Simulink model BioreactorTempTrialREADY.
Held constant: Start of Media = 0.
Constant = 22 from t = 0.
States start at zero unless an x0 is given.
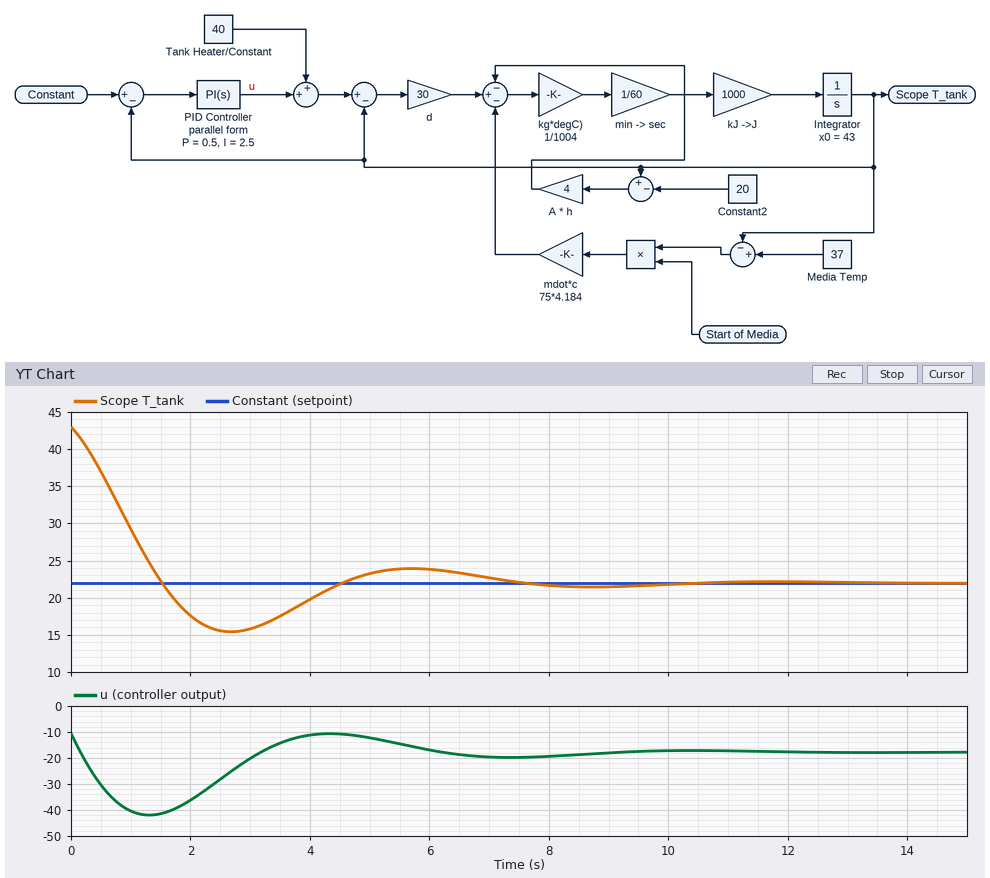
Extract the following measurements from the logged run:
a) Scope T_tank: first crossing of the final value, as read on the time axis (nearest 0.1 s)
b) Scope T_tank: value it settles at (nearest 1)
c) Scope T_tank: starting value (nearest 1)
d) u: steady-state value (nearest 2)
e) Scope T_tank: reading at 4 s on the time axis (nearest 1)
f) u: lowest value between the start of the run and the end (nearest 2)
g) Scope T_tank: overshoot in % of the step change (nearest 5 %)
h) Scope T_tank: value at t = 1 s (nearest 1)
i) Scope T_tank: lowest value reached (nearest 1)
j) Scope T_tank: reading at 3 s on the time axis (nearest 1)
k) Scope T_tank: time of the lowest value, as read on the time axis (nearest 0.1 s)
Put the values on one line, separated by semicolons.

1.5 s; 22; 43; -18; 20; -42; 30 %; 29; 15; 16; 2.7 s
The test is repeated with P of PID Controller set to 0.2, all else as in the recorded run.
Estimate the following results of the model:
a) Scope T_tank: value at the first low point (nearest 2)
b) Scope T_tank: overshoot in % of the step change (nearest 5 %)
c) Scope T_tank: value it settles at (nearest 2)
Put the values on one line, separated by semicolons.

14; 40 %; 22
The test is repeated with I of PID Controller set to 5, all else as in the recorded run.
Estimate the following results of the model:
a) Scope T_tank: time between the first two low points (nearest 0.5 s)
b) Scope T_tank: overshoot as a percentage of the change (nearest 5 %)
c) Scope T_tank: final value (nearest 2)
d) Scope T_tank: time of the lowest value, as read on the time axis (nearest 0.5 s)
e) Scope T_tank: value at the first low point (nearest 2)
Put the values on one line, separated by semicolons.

4.0 s; 45 %; 22; 2.0 s; 12
